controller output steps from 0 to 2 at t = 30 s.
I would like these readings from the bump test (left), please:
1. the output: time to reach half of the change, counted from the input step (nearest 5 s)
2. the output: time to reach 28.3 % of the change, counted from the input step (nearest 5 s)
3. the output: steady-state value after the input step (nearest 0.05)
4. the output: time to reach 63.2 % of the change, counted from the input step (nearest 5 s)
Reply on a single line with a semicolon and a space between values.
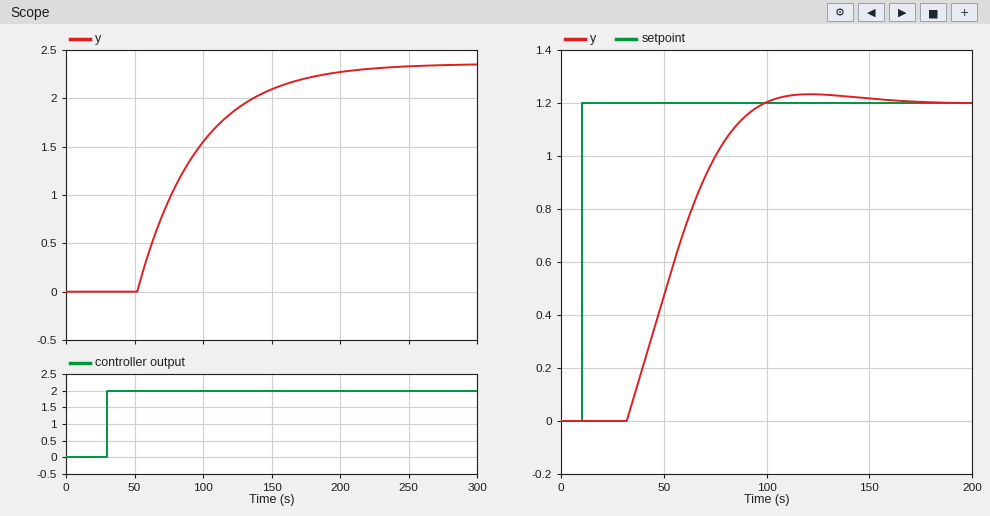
55 s; 35 s; 2.35; 65 s
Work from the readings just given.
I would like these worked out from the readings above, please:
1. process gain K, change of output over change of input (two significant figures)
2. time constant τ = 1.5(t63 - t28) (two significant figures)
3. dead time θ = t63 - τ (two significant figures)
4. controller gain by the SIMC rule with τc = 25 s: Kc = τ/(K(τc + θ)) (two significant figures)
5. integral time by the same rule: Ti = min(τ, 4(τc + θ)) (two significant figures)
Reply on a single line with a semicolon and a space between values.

1.2; 45 s; 20 s; 0.83; 45 s
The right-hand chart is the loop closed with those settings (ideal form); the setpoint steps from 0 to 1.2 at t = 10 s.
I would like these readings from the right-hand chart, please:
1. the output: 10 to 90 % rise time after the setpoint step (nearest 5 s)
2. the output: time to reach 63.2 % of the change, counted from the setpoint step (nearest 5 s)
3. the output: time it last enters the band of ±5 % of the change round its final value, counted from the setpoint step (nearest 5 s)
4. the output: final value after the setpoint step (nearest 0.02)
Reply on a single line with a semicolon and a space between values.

45 s; 50 s; 80 s; 1.20
